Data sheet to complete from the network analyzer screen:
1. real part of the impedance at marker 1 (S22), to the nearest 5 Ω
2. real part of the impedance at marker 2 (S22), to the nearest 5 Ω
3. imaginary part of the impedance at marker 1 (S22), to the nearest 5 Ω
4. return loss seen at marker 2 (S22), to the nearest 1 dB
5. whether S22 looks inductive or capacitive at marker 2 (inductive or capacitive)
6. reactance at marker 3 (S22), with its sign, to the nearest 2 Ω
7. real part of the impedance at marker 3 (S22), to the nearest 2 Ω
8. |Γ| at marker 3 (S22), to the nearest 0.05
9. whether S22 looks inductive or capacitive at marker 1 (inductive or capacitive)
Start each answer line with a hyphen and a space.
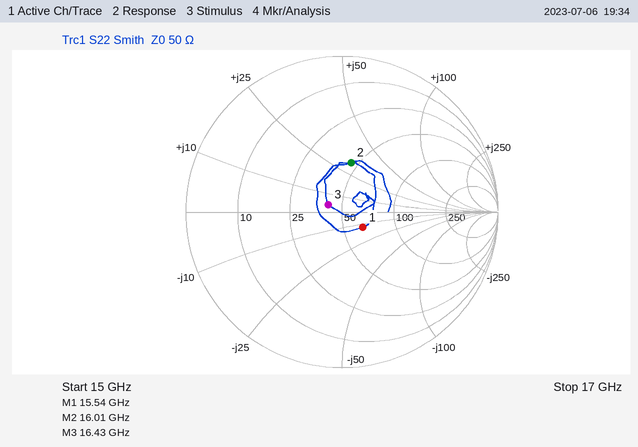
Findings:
- 65 Ω
- 45 Ω
- -15 Ω
- 10 dB
- inductive
- +4 Ω
- 42 Ω
- 0.10
- capacitive
